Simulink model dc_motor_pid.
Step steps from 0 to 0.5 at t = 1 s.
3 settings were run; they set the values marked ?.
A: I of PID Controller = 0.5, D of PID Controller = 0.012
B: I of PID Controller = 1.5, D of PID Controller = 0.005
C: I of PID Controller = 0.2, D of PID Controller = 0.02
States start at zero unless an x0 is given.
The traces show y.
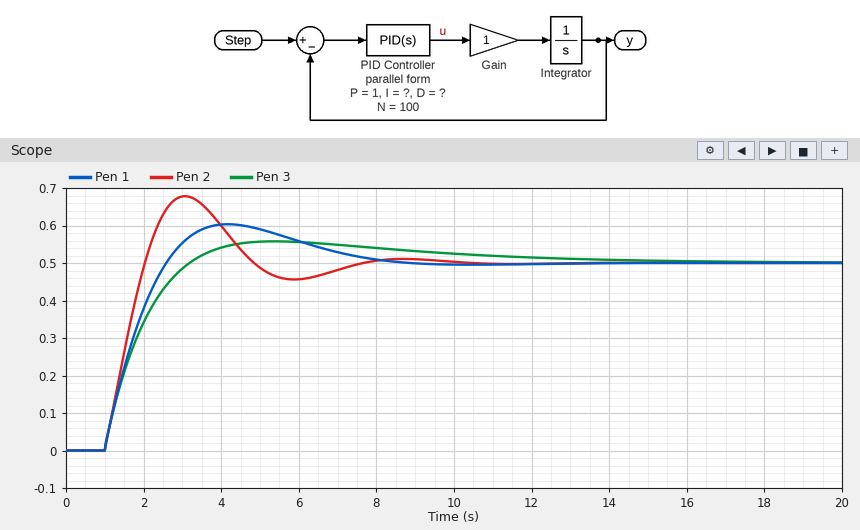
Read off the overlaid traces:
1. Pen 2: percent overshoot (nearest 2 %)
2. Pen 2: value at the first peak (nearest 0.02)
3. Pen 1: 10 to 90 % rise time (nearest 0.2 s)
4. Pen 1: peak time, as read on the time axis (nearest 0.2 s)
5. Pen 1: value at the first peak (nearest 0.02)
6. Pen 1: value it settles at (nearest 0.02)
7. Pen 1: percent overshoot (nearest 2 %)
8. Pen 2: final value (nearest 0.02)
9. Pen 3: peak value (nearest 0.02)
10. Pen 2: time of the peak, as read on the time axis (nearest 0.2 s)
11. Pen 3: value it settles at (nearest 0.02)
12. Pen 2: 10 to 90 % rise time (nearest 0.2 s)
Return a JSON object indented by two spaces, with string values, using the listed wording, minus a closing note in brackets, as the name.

{
  "Pen 2: percent overshoot": "36 %",
  "Pen 2: value at the first peak": "0.68",
  "Pen 1: 10 to 90 % rise time": "1.2 s",
  "Pen 1: peak time, as read on the time axis": "4.2 s",
  "Pen 1: value at the first peak": "0.60",
  "Pen 1: value it settles at": "0.50",
  "Pen 1: percent overshoot": "20 %",
  "Pen 2: final value": "0.50",
  "Pen 3: peak value": "0.56",
  "Pen 2: time of the peak, as read on the time axis": "3.0 s",
  "Pen 3: value it settles at": "0.50",
  "Pen 2: 10 to 90 % rise time": "0.8 s"
}
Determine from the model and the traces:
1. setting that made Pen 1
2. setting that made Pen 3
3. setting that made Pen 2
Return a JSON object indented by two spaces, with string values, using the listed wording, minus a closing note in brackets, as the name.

{
  "setting that made Pen 1": "A",
  "setting that made Pen 3": "C",
  "setting that made Pen 2": "B"
}
